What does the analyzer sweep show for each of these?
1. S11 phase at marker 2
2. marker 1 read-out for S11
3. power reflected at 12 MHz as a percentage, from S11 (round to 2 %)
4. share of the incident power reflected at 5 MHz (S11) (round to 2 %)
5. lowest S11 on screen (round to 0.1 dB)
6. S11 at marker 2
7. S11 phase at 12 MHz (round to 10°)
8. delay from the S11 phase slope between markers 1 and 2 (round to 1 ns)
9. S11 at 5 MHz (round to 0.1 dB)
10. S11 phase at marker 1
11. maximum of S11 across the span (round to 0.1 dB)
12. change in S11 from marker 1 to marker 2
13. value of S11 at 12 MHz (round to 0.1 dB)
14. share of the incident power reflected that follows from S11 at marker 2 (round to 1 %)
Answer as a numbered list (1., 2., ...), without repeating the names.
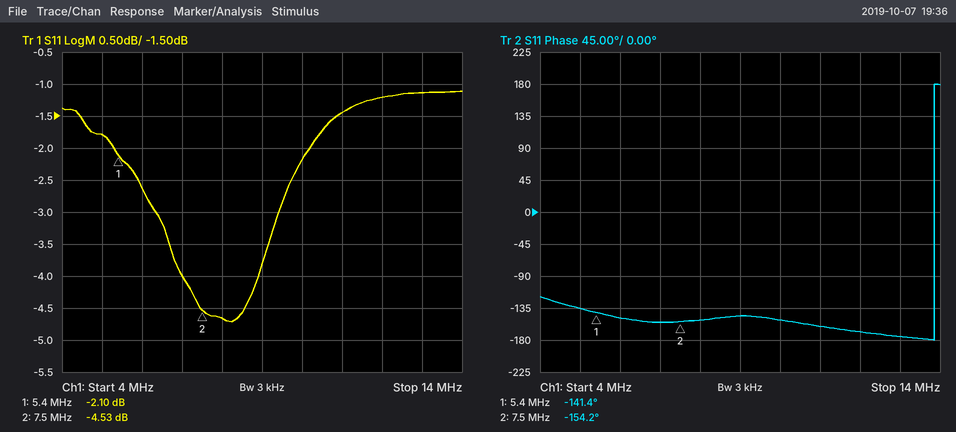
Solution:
1. -154.2°
2. -2.10 dB
3. 76 %
4. 66 %
5. -4.7 dB
6. -4.53 dB
7. -170°
8. 17 ns
9. -1.8 dB
10. -141.4°
11. -1.1 dB
12. -2.43 dB
13. -1.2 dB
14. 35 %
